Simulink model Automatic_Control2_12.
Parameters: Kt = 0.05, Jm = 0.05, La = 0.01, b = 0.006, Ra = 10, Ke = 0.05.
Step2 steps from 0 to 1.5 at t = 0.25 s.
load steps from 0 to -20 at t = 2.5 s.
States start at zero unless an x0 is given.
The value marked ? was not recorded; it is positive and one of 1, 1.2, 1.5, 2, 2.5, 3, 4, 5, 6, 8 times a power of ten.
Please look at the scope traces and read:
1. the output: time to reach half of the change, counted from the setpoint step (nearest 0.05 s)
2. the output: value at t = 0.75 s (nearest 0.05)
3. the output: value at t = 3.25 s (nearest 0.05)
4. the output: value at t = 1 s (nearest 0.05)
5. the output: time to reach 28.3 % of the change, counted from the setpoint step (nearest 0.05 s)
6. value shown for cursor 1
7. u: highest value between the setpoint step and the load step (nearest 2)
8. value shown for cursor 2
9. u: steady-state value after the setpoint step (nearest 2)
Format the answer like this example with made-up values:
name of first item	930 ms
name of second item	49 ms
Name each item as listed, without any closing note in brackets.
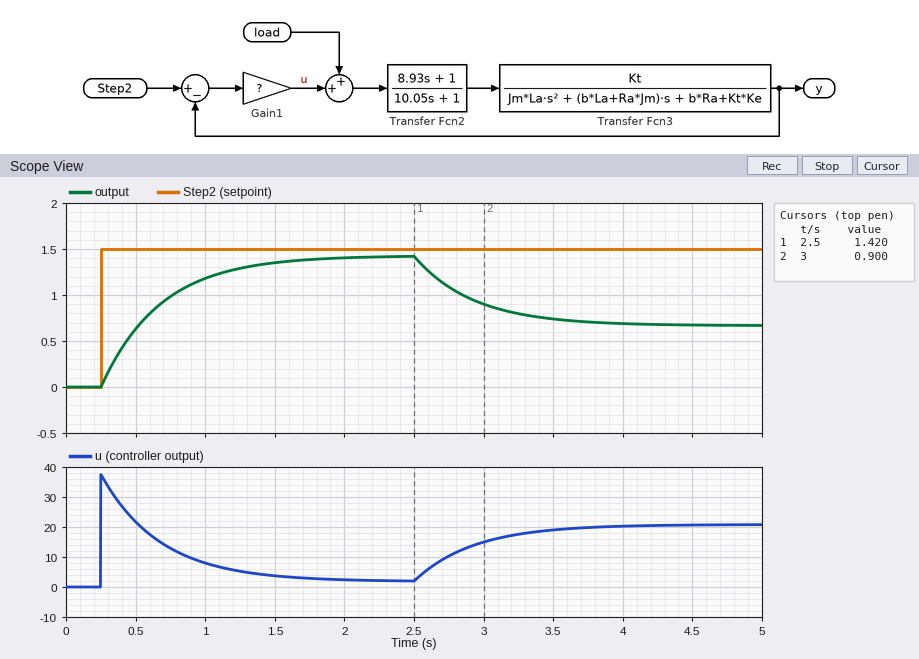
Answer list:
the output: time to reach half of the change, counted from the setpoint step	0.30 s
the output: value at t = 0.75 s	1.00
the output: value at t = 3.25 s	0.80
the output: value at t = 1 s	1.20
the output: time to reach 28.3 % of the change, counted from the setpoint step	0.15 s
value shown for cursor 1	1.420
u: highest value between the setpoint step and the load step	38
value shown for cursor 2	0.900
u: steady-state value after the setpoint step	2
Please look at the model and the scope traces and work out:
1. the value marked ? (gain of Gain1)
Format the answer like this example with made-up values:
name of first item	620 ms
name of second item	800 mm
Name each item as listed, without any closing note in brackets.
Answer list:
the value marked ?	25
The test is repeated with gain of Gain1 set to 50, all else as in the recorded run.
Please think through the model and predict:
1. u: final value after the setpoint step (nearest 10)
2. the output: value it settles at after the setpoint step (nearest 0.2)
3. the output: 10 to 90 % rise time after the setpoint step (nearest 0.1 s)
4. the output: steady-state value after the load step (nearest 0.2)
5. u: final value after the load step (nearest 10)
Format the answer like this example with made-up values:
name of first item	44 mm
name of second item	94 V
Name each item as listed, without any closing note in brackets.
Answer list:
u: final value after the setpoint step	0
the output: value it settles at after the setpoint step	1.4
the output: 10 to 90 % rise time after the setpoint step	0.5 s
the output: steady-state value after the load step	1.0
u: final value after the load step	20
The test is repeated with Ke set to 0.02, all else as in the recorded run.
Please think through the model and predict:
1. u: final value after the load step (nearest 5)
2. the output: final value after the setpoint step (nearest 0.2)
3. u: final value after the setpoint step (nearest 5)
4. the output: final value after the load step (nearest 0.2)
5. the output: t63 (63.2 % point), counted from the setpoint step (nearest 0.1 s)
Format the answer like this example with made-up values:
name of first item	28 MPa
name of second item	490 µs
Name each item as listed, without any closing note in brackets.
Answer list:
u: final value after the load step	20
the output: final value after the setpoint step	1.4
u: final value after the setpoint step	0
the output: final value after the load step	0.6
the output: t63 (63.2 % point), counted from the setpoint step	0.4 s
